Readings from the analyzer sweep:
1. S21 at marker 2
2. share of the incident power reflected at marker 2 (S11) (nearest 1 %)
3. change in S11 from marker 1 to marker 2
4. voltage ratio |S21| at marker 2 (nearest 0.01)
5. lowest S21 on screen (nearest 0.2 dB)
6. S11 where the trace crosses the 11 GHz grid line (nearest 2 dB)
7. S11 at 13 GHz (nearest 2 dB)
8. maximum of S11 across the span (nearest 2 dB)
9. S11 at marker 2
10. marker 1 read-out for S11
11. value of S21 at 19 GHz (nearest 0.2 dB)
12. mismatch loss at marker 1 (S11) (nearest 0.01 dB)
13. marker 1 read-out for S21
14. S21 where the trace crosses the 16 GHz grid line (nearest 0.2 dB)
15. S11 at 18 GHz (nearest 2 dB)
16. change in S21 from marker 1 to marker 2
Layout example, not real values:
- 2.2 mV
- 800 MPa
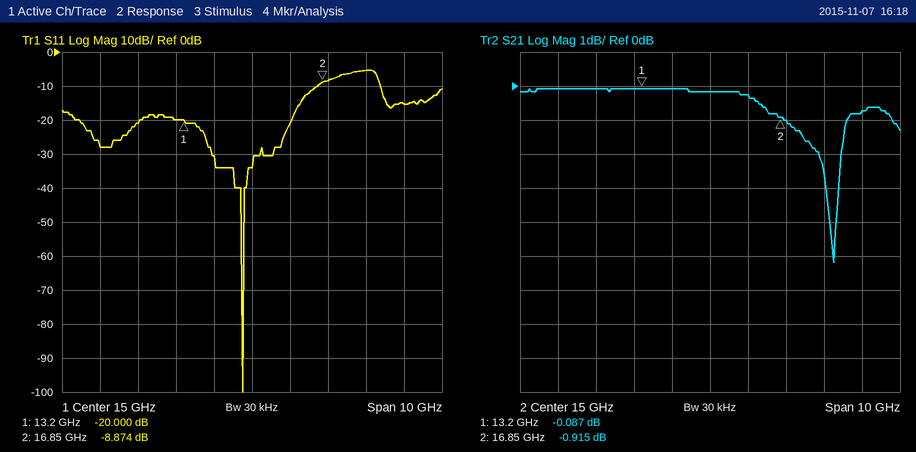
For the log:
- -0.915 dB
- 13 %
- 11.126 dB
- 0.90
- -5.2 dB
- -28 dB
- -20 dB
- -6 dB
- -8.874 dB
- -20.000 dB
- -0.8 dB
- 0.04 dB
- -0.087 dB
- -0.2 dB
- -6 dB
- -0.828 dB
